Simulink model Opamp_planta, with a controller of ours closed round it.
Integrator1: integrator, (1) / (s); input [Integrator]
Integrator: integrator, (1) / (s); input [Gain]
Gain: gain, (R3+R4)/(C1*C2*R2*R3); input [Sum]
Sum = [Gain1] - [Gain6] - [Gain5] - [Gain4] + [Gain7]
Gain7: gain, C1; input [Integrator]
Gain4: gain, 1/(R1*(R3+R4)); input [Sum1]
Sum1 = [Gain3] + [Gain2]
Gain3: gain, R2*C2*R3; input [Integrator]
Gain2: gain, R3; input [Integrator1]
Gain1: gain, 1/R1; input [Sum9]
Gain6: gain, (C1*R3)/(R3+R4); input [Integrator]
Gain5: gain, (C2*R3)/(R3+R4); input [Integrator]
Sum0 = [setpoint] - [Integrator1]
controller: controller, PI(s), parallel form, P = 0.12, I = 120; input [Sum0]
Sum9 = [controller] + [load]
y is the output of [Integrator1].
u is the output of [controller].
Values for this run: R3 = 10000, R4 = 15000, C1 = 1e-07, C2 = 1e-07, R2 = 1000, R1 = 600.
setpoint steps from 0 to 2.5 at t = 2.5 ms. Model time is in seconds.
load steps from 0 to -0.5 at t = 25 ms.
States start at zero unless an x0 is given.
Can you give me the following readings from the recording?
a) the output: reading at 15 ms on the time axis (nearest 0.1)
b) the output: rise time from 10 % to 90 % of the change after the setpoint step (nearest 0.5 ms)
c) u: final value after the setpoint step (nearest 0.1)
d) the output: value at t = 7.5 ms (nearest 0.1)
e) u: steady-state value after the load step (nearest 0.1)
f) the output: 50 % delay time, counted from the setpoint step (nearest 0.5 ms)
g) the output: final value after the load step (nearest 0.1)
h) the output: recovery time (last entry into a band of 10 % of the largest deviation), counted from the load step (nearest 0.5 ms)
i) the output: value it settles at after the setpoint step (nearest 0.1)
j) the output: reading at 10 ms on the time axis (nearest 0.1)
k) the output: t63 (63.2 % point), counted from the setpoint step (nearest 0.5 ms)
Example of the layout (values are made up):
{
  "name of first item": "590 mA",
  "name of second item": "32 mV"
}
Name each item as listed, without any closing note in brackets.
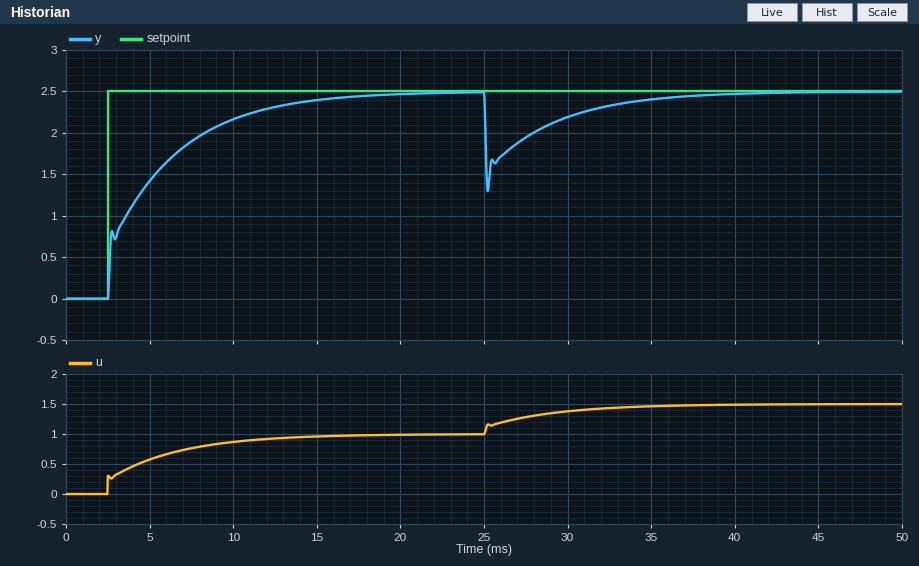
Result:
{
  "the output: reading at 15 ms on the time axis": "2.4",
  "the output: rise time from 10 % to 90 % of the change after the setpoint step": "8.5 ms",
  "u: final value after the setpoint step": "1.0",
  "the output: value at t = 7.5 ms": "1.9",
  "u: steady-state value after the load step": "1.5",
  "the output: 50 % delay time, counted from the setpoint step": "2.0 ms",
  "the output: final value after the load step": "2.5",
  "the output: recovery time (last entry into a band of 10 % of the largest deviation), counted from the load step": "9.0 ms",
  "the output: value it settles at after the setpoint step": "2.5",
  "the output: reading at 10 ms on the time axis": "2.2",
  "the output: t63 (63.2 % point), counted from the setpoint step": "3.0 ms"
}
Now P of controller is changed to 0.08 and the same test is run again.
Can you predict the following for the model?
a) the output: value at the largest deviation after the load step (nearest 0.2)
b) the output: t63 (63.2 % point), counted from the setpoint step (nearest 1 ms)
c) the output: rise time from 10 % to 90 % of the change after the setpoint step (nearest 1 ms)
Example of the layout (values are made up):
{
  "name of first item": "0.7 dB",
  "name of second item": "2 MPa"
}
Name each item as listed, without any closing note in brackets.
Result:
{
  "the output: value at the largest deviation after the load step": "1.2",
  "the output: t63 (63.2 % point), counted from the setpoint step": "3 ms",
  "the output: rise time from 10 % to 90 % of the change after the setpoint step": "8 ms"
}
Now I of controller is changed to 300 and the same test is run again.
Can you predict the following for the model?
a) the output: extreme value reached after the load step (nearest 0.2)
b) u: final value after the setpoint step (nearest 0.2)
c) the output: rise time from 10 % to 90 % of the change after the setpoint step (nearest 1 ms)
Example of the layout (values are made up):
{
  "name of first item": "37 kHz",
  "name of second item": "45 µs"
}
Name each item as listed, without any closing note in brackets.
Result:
{
  "the output: extreme value reached after the load step": "1.4",
  "u: final value after the setpoint step": "1.0",
  "the output: rise time from 10 % to 90 % of the change after the setpoint step": "3 ms"
}
